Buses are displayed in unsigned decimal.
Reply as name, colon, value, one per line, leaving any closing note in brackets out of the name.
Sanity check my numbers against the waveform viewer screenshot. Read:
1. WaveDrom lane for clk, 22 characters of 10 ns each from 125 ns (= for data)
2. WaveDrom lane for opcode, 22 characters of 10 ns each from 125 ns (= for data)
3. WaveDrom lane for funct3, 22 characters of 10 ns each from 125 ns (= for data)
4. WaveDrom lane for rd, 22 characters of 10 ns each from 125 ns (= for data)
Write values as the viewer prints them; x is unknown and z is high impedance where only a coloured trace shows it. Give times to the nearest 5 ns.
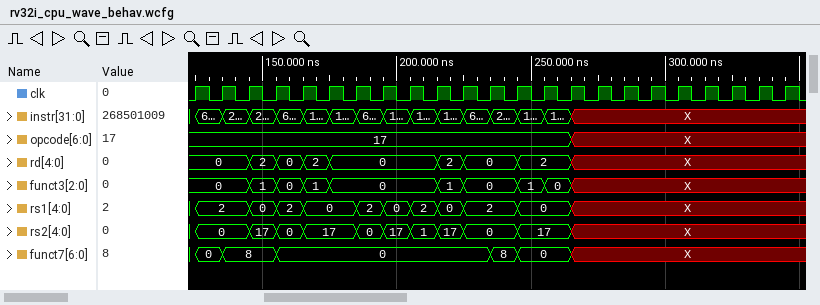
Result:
WaveDrom lane for clk, 22 characters of 10 ns each from 125 ns: {name: 'clk', wave: 'p.....................'}
WaveDrom lane for opcode, 22 characters of 10 ns each from 125 ns: {name: 'opcode', wave: '=.............x.......', data: '17'}
WaveDrom lane for funct3, 22 characters of 10 ns each from 125 ns: {name: 'funct3', wave: '=.====...==.==x.......', data: '0 1 0 1 0 1 0 1 0'}
WaveDrom lane for rd, 22 characters of 10 ns each from 125 ns: {name: 'rd', wave: '=.====...==.=.x.......', data: '0 2 0 2 0 2 0 2'}
